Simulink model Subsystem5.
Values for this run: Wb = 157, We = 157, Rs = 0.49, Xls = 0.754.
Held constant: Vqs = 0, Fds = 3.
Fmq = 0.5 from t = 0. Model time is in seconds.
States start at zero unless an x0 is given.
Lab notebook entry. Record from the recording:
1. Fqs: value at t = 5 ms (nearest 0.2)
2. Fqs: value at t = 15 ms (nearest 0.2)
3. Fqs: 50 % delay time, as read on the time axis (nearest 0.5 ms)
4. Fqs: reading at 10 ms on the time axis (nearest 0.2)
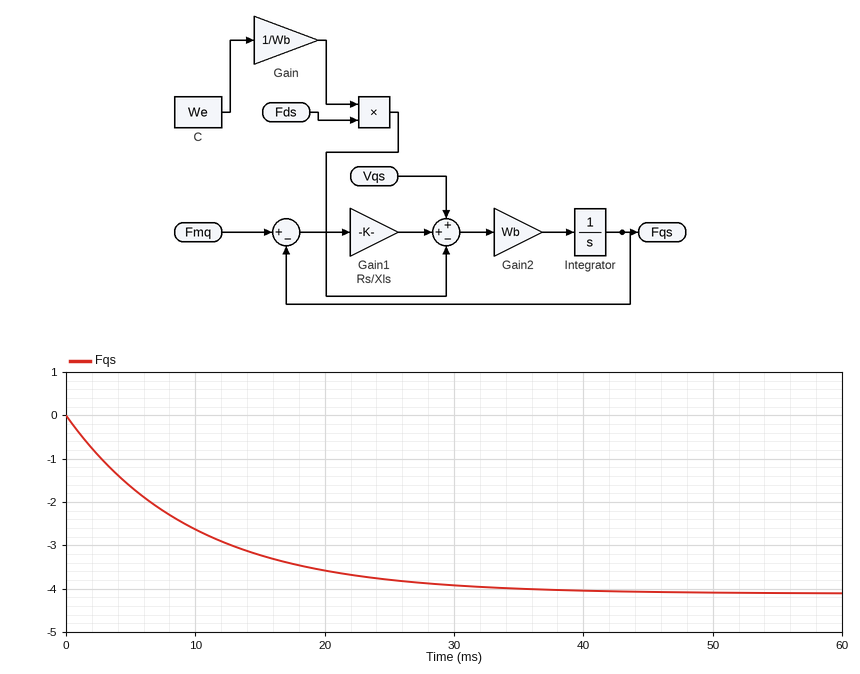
-1.6
-3.2
7.0 ms
-2.6
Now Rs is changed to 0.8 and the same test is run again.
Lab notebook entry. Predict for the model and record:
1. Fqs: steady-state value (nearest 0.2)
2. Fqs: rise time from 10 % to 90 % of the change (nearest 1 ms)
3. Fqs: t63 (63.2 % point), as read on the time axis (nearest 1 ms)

-2.4
13 ms
6 ms
